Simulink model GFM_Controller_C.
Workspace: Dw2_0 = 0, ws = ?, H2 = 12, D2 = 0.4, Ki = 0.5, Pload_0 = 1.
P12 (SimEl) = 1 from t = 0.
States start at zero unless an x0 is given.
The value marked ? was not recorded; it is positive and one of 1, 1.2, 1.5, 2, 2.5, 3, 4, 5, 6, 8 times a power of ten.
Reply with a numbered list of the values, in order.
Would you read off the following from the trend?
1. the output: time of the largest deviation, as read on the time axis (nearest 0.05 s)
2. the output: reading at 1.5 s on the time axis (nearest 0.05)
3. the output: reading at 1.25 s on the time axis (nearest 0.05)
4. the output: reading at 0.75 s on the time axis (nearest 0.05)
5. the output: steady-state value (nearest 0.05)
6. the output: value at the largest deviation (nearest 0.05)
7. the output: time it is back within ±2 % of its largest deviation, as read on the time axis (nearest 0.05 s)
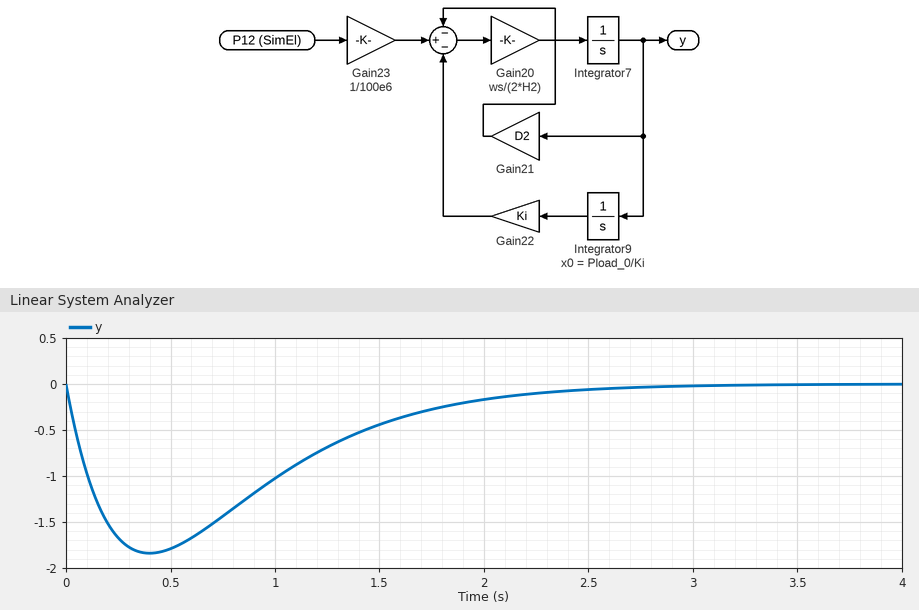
1. 0.40 s
2. -0.45
3. -0.70
4. -1.45
5. 0.00
6. -1.85
7. 2.75 s
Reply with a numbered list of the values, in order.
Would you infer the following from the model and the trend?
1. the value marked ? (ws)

1. 300
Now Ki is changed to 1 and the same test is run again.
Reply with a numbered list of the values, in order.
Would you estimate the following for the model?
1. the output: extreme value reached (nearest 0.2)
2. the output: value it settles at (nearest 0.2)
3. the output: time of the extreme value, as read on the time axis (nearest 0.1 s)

1. -1.6
2. 0.0
3. 0.3 s
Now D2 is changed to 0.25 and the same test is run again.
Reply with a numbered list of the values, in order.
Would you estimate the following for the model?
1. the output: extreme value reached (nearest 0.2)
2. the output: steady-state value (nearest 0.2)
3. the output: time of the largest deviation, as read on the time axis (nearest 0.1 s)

1. -2.4
2. 0.0
3. 0.5 s
